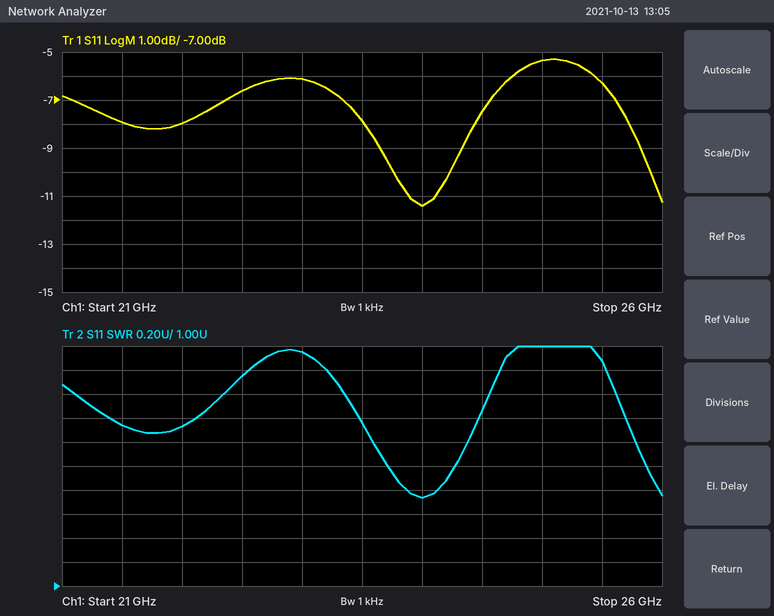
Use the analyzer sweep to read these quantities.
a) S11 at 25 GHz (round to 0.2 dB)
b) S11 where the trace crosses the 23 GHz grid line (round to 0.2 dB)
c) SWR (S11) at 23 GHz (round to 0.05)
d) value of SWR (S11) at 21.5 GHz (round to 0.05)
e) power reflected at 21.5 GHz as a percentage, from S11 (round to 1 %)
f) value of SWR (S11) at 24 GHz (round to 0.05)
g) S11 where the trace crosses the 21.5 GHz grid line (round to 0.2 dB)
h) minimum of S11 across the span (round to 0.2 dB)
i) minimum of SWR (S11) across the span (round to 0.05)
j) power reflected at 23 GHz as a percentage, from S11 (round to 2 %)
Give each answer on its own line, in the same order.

-5.4 dB
-6.2 dB
2.95
2.35
16 %
1.75
-8.0 dB
-11.4 dB
1.75
24 %
